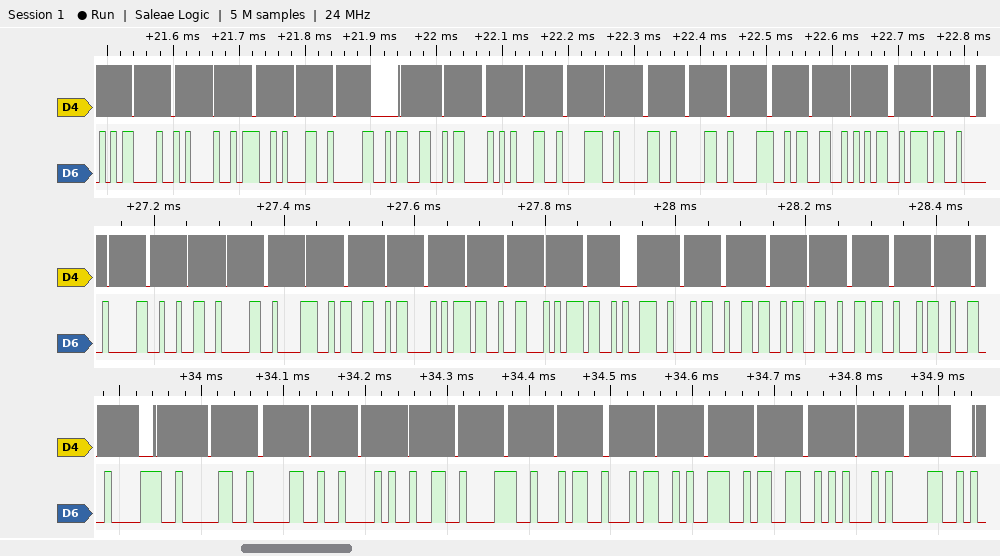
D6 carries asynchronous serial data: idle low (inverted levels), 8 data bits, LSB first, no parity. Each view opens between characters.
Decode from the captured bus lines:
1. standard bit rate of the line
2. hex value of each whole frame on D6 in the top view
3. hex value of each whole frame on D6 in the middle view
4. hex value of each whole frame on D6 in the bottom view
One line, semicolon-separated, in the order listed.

115200 baud; E5, EB, 8B, 9D, 9F, 99, 79, 9D, 8F, 9F, 9F, 8F, 99, 95, 91; 9F, 9B, 9F, 8F, 99, 79, 91, 73, 91, 8D, 97, 93, 99, 93, 97; 8F, 9F, 9F, 7B, 9B, 8F, 97, 97, 8D, 99, 75, 9F
